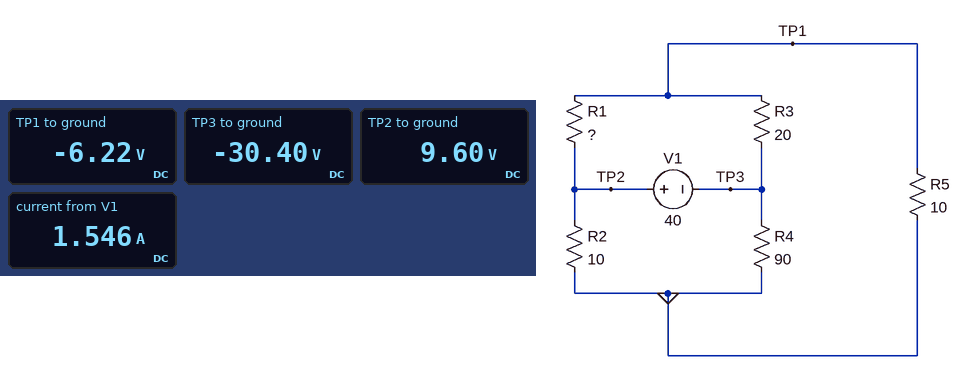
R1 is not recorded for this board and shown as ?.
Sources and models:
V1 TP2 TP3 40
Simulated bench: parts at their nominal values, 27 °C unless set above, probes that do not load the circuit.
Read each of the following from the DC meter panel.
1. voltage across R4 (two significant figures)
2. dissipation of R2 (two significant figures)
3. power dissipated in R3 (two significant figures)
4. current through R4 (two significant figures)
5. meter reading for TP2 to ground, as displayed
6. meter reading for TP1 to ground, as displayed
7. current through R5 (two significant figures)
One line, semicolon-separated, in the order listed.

30 V; 9.2 W; 29 W; 340 mA; 9.60 V; -6.22 V; 620 mA
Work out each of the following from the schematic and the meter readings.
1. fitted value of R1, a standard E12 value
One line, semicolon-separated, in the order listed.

27 Ω
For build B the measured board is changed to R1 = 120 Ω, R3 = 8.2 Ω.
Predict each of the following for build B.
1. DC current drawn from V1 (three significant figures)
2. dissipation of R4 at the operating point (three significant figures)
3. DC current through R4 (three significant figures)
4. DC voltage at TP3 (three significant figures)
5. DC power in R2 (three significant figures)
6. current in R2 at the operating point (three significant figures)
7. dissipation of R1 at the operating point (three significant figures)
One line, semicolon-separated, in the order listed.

1.76 A; 6.79 W; 275 mA; -24.7 V; 23.4 W; 1.53 A; 6.45 W
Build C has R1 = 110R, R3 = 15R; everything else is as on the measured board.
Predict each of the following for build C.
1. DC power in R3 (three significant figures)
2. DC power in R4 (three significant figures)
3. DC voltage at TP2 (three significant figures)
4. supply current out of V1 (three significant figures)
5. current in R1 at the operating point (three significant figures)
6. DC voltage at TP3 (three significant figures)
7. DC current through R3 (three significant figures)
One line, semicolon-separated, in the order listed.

20.6 W; 8.27 W; 12.7 V; 1.48 A; 204 mA; -27.3 V; 1.17 A
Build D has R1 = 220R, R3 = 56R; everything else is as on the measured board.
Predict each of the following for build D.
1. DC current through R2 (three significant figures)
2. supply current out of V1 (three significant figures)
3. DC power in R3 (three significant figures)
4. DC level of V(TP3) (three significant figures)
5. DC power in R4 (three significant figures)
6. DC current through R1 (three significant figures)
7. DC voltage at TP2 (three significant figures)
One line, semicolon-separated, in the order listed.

794 mA; 850 mA; 13.7 W; -32.1 V; 11.4 W; 56.0 mA; 7.94 V
